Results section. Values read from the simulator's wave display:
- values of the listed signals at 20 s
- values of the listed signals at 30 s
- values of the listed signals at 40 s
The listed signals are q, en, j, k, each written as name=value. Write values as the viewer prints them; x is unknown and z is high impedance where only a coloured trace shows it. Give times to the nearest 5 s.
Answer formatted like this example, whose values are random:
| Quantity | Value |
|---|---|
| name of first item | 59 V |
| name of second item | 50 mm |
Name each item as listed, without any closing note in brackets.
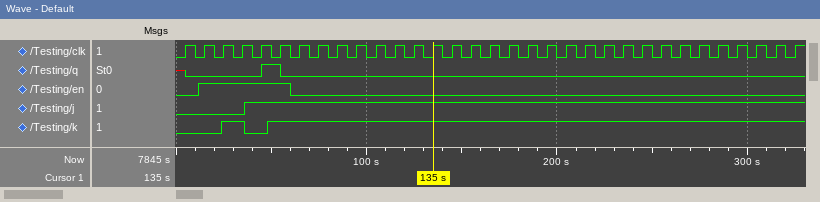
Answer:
| Quantity | Value |
|---|---|
| values of the listed signals at 20 s | q=0, en=1, j=0, k=0 |
| values of the listed signals at 30 s | q=0, en=1, j=0, k=1 |
| values of the listed signals at 40 s | q=0, en=1, j=1, k=0 |
